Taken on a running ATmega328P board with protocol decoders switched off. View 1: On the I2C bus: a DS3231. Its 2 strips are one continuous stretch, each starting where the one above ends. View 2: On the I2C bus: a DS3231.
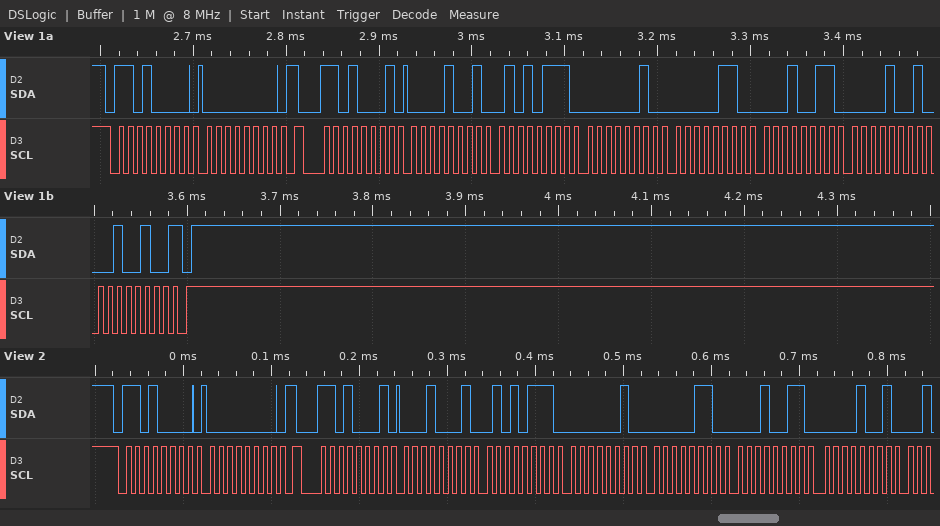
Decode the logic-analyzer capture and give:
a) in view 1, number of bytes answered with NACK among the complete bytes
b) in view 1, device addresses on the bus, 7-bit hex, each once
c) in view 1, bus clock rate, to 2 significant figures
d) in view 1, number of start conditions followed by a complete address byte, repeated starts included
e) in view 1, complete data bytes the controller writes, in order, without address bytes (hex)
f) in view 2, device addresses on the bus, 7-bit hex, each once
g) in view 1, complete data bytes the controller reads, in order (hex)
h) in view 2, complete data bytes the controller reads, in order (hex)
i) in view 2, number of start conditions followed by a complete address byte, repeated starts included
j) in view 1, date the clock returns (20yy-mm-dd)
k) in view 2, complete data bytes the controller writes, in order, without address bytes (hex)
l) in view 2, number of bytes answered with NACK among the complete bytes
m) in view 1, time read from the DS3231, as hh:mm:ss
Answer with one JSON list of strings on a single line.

["1", "0x68", "100 kHz", "2", "00", "0x68", "09 57 02 06 13 09 24", "11 57 02 06 13 09", "2", "2024-09-13", "00", "0", "02:57:09"]
